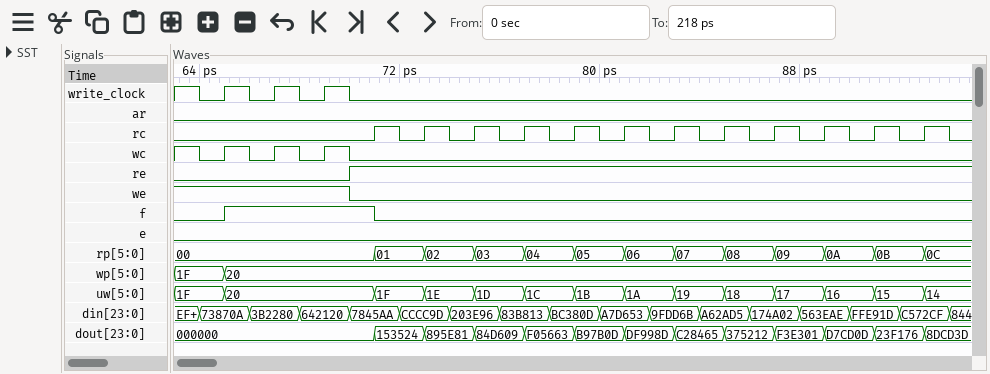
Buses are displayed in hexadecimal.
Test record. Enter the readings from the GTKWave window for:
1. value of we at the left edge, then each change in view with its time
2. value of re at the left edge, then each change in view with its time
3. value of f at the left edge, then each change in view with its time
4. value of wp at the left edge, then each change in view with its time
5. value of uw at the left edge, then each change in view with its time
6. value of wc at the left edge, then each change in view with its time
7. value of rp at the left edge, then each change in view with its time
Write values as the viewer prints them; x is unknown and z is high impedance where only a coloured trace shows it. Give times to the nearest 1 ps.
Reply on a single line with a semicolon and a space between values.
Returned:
1, 0 at 70 ps; 0, 1 at 70 ps; 0, 1 at 65 ps, 0 at 71 ps; 1F, 20 at 65 ps; 1F, 20 at 65 ps, 1F at 71 ps, 1E at 73 ps, 1D at 75 ps, 1C at 77 ps, 1B at 79 ps, 1A at 81 ps, 19 at 83 ps, 18 at 85 ps, 17 at 87 ps, 16 at 89 ps, 15 at 91 ps, 14 at 93 ps; 1, 0 at 64 ps, 1 at 65 ps, 0 at 66 ps, 1 at 67 ps, 0 at 68 ps, 1 at 69 ps, 0 at 70 ps; 00, 01 at 71 ps, 02 at 73 ps, 03 at 75 ps, 04 at 77 ps, 05 at 79 ps, 06 at 81 ps, 07 at 83 ps, 08 at 85 ps, 09 at 87 ps, 0A at 89 ps, 0B at 91 ps, 0C at 93 ps
